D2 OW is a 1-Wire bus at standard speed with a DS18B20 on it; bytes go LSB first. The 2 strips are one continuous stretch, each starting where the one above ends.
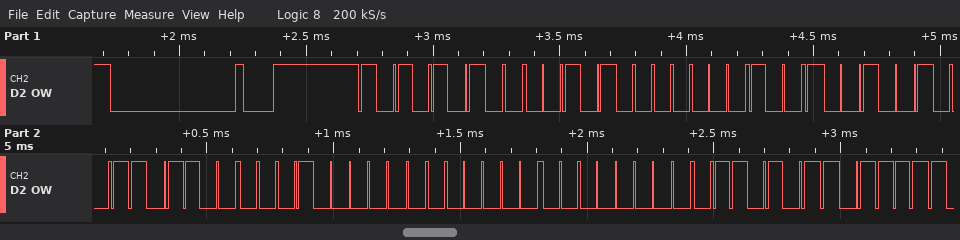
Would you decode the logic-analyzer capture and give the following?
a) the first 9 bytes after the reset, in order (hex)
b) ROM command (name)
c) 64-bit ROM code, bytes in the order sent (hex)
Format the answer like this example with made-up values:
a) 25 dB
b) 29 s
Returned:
a) 55 28 20 49 36 08 00 00 D6
b) Match ROM
c) 28 20 49 36 08 00 00 D6
